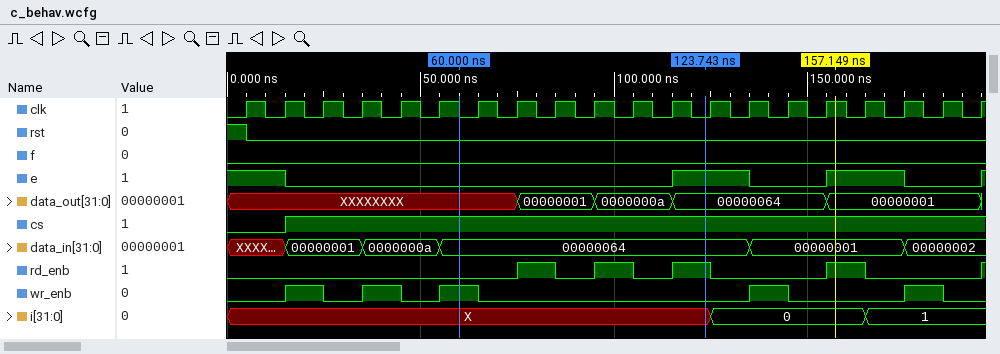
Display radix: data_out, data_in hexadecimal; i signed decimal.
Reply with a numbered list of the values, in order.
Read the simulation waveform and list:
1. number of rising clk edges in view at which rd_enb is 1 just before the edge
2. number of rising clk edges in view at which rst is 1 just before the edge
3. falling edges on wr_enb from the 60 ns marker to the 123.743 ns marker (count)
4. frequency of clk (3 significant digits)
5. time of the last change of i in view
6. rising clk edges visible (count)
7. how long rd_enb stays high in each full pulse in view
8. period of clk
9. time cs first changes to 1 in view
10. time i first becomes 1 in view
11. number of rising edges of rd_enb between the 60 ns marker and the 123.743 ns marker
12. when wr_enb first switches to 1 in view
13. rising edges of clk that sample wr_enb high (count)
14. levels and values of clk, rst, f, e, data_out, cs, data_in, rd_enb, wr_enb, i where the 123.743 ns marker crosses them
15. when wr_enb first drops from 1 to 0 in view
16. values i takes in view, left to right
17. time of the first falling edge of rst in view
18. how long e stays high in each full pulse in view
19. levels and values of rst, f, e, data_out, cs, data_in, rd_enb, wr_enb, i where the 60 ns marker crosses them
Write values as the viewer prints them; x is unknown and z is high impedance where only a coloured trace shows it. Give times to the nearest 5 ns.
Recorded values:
1. 4
2. 1
3. 1
4. 100 MHz
5. 165 ns
6. 20
7. 10 ns, 10 ns, 10 ns, 10 ns
8. 10 ns
9. 15 ns
10. 165 ns
11. 3
12. 15 ns
13. 5
14. clk=0, rst=0, f=0, e=1, data_out=00000064, cs=1, data_in=00000064, rd_enb=1, wr_enb=0, i=X
15. 25 ns
16. X, 0, 1
17. 5 ns
18. 20 ns, 20 ns
19. rst=0, f=0, e=0, data_out=XXXXXXXX, cs=1, data_in=00000064, rd_enb=0, wr_enb=1, i=X
